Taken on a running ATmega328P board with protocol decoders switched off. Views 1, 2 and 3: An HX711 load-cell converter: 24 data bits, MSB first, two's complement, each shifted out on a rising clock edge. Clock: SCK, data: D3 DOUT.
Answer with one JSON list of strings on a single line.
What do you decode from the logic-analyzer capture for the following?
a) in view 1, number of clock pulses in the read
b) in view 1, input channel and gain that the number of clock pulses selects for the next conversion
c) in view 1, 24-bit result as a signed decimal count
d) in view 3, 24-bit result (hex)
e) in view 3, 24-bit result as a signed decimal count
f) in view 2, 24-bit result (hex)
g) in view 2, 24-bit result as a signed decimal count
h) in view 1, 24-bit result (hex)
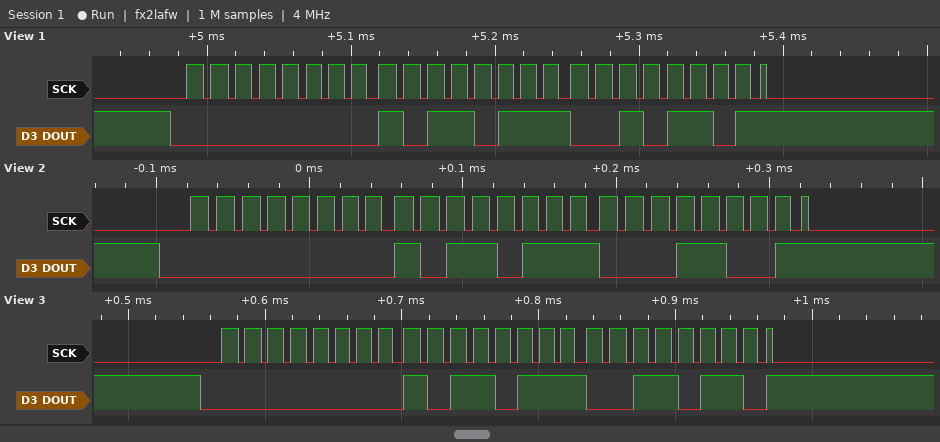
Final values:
["25", "channel A, gain 128", "46893", "0x00B736", "46902", "0x00B719", "46873", "0x00B72D"]
